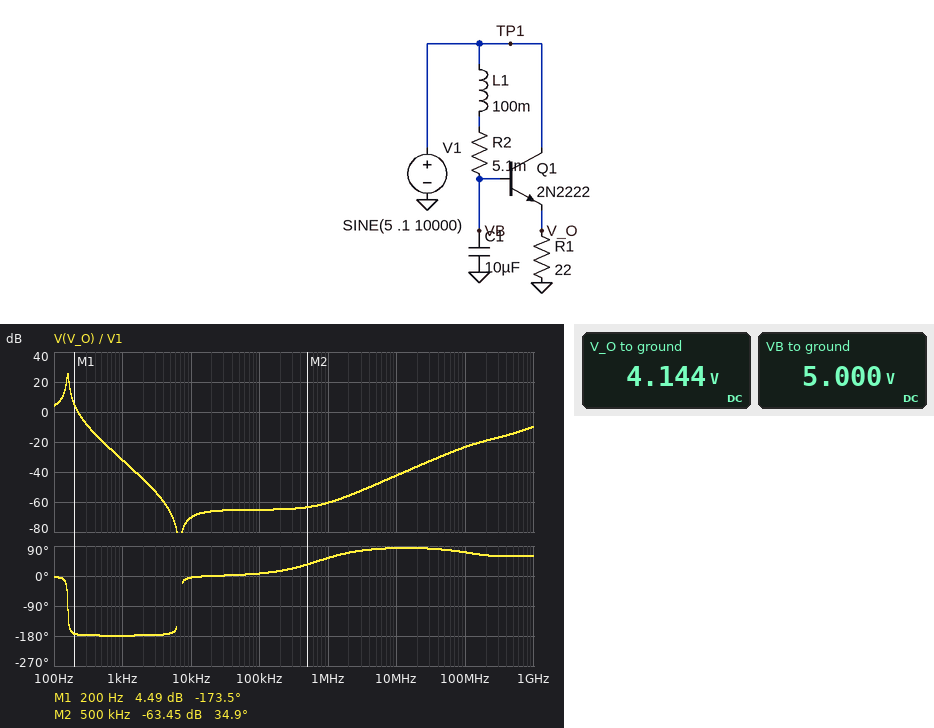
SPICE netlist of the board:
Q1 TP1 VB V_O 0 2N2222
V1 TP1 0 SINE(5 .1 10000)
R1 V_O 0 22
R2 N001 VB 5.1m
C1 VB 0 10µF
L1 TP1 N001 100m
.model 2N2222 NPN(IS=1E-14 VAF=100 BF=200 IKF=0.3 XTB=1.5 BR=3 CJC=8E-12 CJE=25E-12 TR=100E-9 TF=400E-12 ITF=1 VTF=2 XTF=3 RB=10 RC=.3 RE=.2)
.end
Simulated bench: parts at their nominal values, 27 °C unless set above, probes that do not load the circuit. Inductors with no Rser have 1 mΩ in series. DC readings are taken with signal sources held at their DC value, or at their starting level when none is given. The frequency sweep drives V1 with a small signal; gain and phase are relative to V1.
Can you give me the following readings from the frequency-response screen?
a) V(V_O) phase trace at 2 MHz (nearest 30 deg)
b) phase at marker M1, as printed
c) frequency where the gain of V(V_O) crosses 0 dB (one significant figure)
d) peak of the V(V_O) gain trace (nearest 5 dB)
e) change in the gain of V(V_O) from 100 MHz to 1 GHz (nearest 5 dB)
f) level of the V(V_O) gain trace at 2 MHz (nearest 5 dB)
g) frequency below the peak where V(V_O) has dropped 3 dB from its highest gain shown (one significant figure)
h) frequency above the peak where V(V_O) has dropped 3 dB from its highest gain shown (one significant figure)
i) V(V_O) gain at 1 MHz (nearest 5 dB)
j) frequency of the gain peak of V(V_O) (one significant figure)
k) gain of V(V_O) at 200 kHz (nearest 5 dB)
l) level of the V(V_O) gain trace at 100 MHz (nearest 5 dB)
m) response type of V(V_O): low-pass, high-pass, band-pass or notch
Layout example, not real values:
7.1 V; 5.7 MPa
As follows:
60 deg; -173.5 deg; 200 Hz; 25 dB; 15 dB; -55 dB; 200 Hz; 200 Hz; -60 dB; 200 Hz; -65 dB; -25 dB; band-pass
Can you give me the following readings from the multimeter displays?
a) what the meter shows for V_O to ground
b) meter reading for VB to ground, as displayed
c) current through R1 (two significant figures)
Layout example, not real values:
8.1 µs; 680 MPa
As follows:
4.144 V; 5.000 V; 190 mA
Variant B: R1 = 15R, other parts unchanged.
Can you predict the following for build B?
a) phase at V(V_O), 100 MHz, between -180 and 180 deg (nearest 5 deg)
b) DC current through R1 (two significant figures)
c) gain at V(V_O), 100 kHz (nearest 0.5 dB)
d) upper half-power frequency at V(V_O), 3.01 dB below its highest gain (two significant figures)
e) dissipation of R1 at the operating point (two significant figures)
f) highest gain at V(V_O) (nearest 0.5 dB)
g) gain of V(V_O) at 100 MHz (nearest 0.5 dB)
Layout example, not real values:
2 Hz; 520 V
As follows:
55 deg; 270 mA; -62.5 dB; 170 Hz; 1.1 W; 20.5 dB; -20.0 dB
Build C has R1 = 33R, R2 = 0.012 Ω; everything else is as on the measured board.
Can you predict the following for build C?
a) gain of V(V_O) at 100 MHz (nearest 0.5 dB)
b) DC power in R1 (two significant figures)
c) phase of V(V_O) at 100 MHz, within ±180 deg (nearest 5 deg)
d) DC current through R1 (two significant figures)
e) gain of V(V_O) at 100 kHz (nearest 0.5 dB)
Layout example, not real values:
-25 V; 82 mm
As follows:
-25.0 dB; 530 mW; 80 deg; 130 mA; -67.0 dB
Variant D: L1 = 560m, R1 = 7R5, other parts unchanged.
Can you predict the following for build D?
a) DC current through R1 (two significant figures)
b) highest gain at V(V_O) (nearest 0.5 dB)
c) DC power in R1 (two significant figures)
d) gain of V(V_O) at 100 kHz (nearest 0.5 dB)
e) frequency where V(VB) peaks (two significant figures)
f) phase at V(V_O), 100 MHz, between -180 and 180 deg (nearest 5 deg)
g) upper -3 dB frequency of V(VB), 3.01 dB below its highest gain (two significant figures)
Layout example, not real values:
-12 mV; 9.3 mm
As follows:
530 mA; 3.5 dB; 2.1 W; -56.0 dB; 59 Hz; 25 deg; 80 Hz
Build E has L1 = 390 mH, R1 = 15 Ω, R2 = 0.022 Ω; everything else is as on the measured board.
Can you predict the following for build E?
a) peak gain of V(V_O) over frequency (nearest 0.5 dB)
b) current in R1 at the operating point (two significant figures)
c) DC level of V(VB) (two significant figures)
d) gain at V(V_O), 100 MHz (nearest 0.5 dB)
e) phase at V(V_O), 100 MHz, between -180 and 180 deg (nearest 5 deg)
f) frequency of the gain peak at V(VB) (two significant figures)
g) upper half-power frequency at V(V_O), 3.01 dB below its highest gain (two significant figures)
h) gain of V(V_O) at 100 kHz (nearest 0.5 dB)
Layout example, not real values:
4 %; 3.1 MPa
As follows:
14.5 dB; 270 mA; 5.0 V; -20.0 dB; 55 deg; 80 Hz; 87 Hz; -62.5 dB
